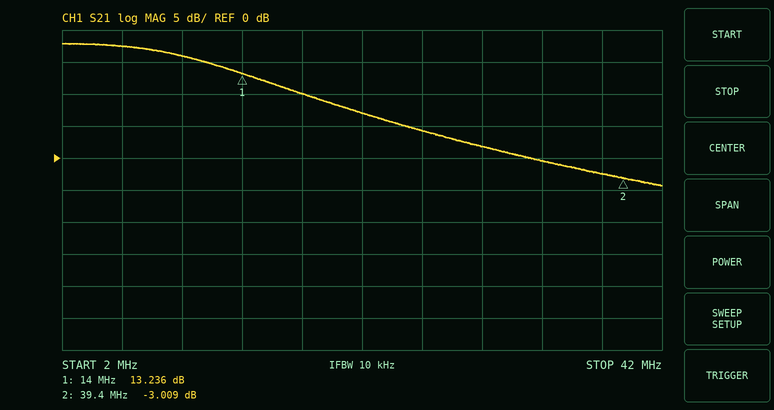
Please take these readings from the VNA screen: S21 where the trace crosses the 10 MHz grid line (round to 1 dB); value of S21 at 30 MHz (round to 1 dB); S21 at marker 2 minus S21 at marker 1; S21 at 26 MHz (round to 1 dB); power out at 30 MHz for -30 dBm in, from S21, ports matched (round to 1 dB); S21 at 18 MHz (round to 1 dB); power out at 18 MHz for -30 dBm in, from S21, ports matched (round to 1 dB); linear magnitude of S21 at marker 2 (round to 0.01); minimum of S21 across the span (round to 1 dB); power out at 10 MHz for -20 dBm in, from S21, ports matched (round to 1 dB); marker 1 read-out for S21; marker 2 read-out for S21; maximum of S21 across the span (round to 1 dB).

16 dB
2 dB
-16.245 dB
4 dB
-28 dBm
10 dB
-20 dBm
0.71
-4 dB
-4 dBm
13.236 dB
-3.009 dB
18 dB
